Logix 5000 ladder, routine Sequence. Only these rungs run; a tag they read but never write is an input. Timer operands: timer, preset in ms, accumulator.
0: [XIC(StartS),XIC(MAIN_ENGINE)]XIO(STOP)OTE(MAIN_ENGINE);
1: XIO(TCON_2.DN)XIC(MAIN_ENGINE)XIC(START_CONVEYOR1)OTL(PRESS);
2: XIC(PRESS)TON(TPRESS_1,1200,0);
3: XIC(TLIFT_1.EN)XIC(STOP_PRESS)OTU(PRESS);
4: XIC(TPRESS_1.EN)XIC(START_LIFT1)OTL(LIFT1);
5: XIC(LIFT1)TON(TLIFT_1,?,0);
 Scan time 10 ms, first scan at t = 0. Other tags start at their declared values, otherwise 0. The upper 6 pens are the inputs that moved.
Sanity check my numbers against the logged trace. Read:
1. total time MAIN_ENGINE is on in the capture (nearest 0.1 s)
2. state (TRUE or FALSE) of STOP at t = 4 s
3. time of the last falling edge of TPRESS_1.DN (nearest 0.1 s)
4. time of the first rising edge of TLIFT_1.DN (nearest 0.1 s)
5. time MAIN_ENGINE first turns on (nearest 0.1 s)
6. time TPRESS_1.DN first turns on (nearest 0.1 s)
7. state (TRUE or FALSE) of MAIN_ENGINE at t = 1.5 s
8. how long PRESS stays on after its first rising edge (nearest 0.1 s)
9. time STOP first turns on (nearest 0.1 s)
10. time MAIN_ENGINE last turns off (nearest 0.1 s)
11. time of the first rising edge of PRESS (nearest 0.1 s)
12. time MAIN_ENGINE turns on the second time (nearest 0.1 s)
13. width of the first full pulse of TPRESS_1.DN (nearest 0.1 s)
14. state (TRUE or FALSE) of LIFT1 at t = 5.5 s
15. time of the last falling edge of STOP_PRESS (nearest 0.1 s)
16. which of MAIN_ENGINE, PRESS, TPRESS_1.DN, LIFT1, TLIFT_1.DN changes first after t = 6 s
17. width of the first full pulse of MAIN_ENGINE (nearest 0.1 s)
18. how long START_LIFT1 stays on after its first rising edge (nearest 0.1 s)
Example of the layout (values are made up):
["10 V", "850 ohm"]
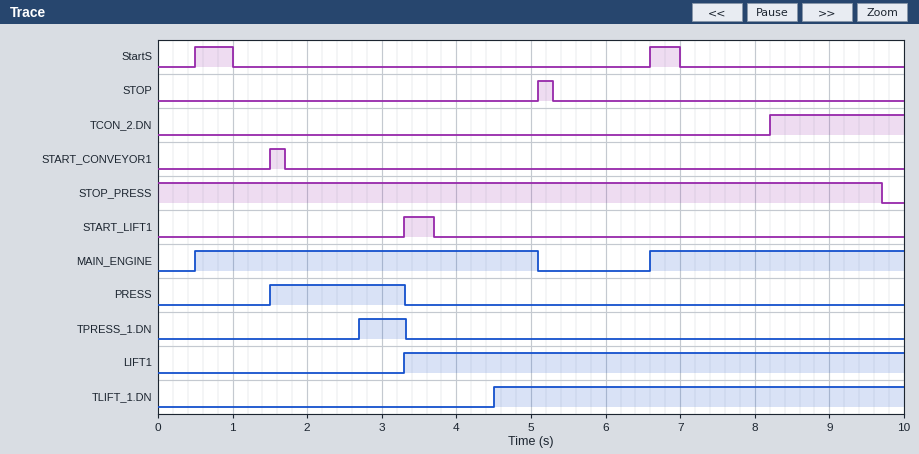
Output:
["8.0 s", "FALSE", "3.3 s", "4.5 s", "0.5 s", "2.7 s", "TRUE", "1.8 s", "5.1 s", "5.1 s", "1.5 s", "6.6 s", "0.6 s", "TRUE", "9.7 s", "MAIN_ENGINE", "4.6 s", "0.4 s"]
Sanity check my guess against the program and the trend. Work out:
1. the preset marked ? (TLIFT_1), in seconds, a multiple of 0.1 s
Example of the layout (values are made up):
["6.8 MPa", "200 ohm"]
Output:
["1.2 s"]
